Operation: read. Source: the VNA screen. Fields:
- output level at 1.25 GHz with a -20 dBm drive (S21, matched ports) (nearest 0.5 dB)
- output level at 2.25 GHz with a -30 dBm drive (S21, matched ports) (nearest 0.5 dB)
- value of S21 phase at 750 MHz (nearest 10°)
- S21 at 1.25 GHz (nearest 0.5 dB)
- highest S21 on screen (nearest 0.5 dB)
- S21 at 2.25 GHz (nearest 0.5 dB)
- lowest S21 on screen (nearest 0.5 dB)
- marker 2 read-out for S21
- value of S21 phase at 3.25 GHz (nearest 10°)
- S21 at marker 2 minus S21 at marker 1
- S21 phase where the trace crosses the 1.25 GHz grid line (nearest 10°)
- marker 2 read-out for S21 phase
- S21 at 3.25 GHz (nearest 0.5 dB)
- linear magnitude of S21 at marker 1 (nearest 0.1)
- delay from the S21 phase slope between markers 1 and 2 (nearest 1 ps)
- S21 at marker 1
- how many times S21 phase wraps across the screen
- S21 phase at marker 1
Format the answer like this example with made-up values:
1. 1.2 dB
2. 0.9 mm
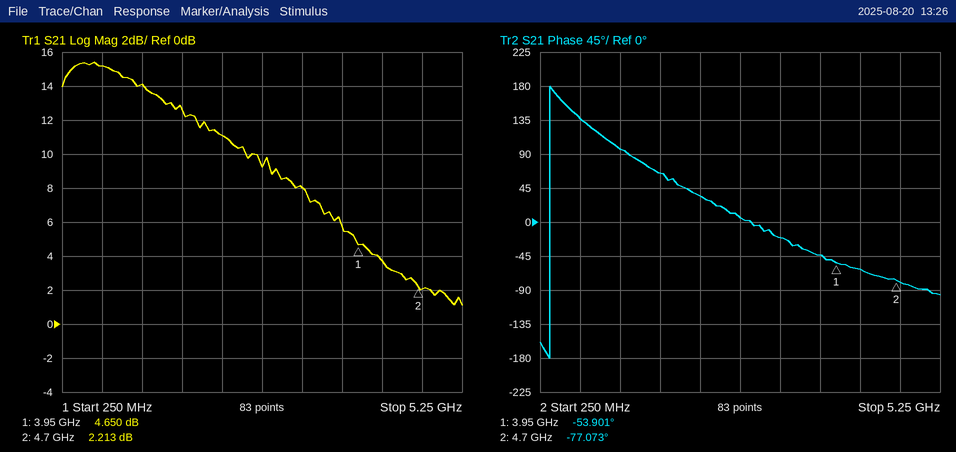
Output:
1. -6.0 dBm
2. -19.0 dBm
3. 140°
4. 14.0 dB
5. 15.5 dB
6. 11.0 dB
7. 1.0 dB
8. 2.213 dB
9. -20°
10. -2.437 dB
11. 100°
12. -77.073°
13. 8.0 dB
14. 1.7
15. 86 ps
16. 4.650 dB
17. 1
18. -53.901°
